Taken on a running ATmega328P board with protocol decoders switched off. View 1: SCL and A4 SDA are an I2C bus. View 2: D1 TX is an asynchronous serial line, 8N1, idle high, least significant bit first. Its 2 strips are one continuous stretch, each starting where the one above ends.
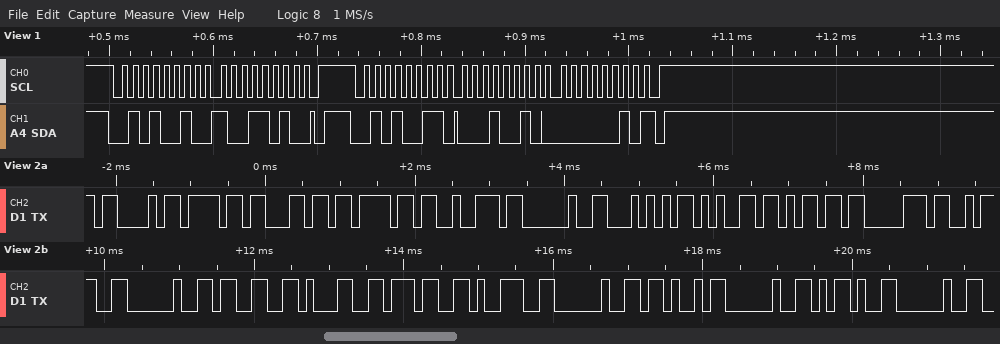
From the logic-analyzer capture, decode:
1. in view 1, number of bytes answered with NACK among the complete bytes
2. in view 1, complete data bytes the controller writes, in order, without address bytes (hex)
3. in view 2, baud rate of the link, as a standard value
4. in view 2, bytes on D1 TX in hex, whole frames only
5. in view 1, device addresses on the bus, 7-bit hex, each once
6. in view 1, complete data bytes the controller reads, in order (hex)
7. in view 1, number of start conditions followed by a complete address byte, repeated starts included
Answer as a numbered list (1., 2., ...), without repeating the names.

1. 1
2. 9A
3. 9600 baud
4. 43 6F 6C 6F 72 20 54 65 6D 70 3A 20 33 31 37 39 20 4B 20 2D 20
5. 0x29
6. 12 02
7. 2
